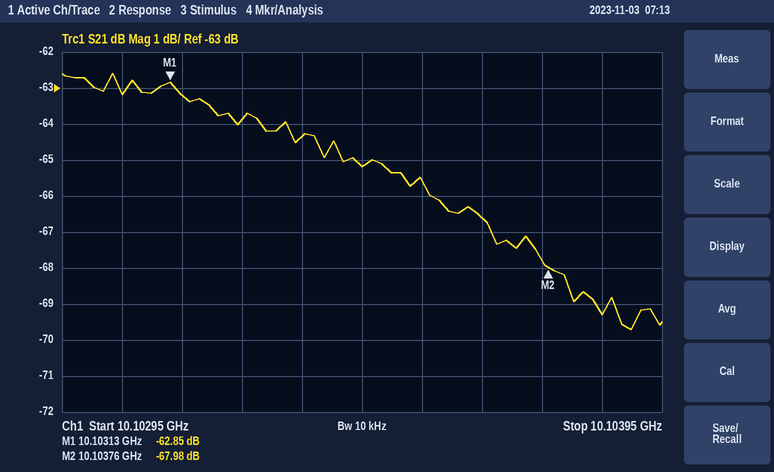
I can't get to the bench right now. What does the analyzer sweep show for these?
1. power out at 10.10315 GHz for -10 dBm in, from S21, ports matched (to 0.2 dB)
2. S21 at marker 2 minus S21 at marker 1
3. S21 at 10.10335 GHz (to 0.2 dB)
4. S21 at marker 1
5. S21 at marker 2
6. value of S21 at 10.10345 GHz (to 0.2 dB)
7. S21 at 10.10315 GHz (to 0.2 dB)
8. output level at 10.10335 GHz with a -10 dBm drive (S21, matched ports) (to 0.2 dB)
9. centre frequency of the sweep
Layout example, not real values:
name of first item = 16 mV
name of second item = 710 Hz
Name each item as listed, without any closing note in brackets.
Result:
power out at 10.10315 GHz for -10 dBm in, from S21, ports matched = -73.2 dBm
S21 at marker 2 minus S21 at marker 1 = -5.13 dB
S21 at 10.10335 GHz = -64.4 dB
S21 at marker 1 = -62.85 dB
S21 at marker 2 = -67.98 dB
value of S21 at 10.10345 GHz = -65.2 dB
S21 at 10.10315 GHz = -63.2 dB
output level at 10.10335 GHz with a -10 dBm drive (S21, matched ports) = -74.4 dBm
centre frequency of the sweep = 10.10345 GHz
